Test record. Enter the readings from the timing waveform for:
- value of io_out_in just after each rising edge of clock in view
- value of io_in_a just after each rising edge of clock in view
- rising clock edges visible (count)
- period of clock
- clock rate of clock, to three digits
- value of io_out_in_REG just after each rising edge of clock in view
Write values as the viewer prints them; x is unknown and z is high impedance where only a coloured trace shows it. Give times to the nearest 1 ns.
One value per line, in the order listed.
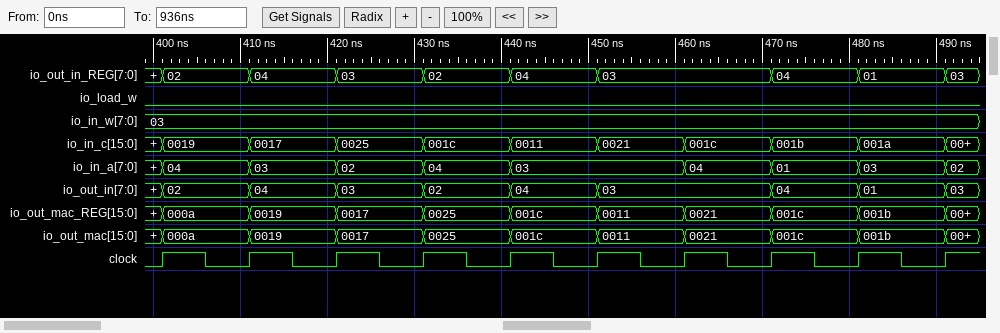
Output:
02, 04, 03, 02, 04, 03, 03, 04, 01, 03
04, 03, 02, 04, 03, 03, 04, 01, 03, 02
10
10 ns
100 MHz
02, 04, 03, 02, 04, 03, 03, 04, 01, 03
